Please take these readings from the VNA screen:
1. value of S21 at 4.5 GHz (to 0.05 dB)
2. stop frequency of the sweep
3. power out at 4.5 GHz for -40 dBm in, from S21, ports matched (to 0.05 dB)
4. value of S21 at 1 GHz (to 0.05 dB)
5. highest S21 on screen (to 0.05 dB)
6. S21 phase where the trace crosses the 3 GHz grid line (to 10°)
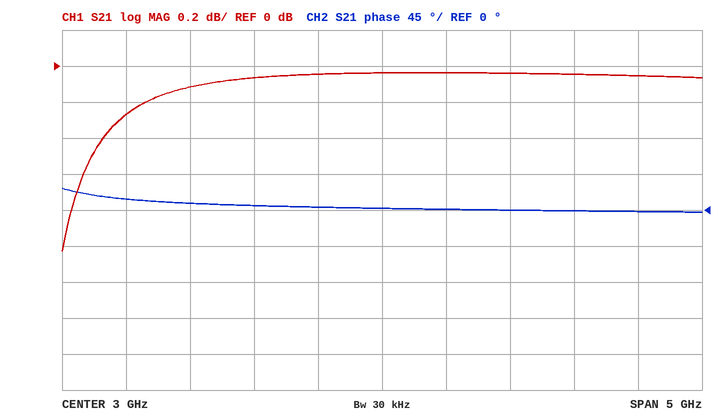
-0.05 dB
5.5 GHz
-40.05 dBm
-0.25 dB
-0.05 dB
0°
